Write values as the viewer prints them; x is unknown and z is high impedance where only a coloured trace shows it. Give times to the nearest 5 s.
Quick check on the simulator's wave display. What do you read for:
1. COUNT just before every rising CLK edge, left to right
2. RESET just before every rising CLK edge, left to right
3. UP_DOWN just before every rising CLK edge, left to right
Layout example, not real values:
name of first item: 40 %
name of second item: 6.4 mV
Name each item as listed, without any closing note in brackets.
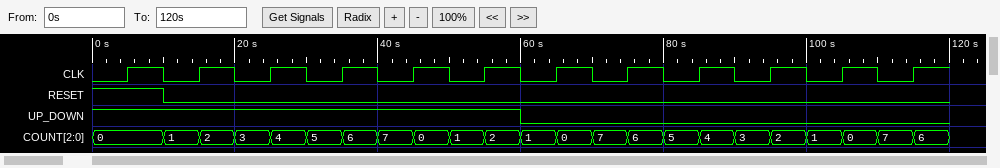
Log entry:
COUNT just before every rising CLK edge, left to right: 0, 1, 3, 5, 7, 1, 1, 7, 5, 3, 1, 7
RESET just before every rising CLK edge, left to right: 1 0 0 0 0 0 0 0 0 0 0 0
UP_DOWN just before every rising CLK edge, left to right: 1 1 1 1 1 1 0 0 0 0 0 0
